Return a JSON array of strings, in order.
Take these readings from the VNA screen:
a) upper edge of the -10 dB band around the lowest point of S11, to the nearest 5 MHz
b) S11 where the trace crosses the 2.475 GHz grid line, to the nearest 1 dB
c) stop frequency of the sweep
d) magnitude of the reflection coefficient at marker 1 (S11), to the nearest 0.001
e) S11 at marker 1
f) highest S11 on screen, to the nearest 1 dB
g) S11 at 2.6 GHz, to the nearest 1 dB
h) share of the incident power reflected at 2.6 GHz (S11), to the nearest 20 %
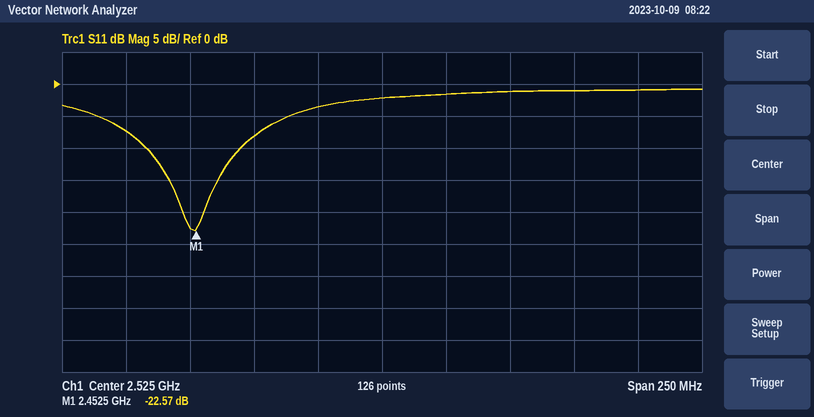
["2.470 GHz", "-8 dB", "2.65 GHz", "0.074", "-22.57 dB", "-1 dB", "-1 dB", "80 %"]
